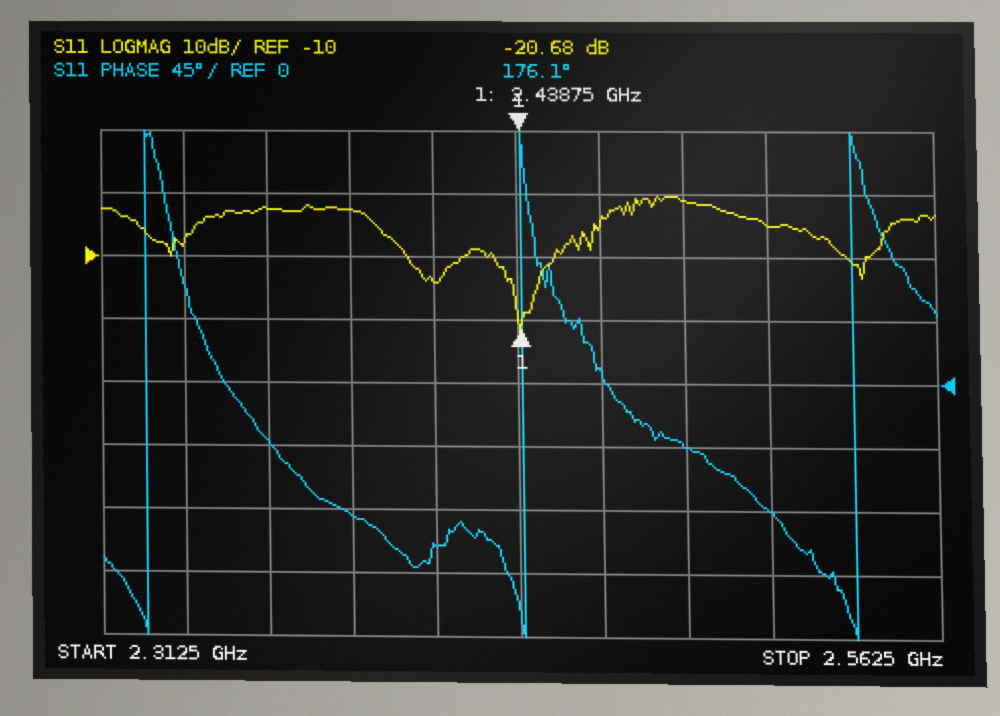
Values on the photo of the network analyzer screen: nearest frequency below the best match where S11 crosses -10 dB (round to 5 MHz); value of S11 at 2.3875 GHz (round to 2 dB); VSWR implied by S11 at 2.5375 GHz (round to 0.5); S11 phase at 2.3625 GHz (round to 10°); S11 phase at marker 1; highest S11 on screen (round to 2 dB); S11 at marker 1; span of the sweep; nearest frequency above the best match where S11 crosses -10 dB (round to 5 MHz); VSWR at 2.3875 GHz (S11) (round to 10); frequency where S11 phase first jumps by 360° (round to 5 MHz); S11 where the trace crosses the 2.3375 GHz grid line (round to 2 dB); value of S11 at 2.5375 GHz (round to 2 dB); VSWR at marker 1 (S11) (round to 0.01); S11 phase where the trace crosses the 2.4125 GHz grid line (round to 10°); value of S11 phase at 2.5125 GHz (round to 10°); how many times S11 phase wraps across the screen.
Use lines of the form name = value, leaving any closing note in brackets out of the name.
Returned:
nearest frequency below the best match where S11 crosses -10 dB = 2.430 GHz
value of S11 at 2.3875 GHz = -2 dB
VSWR implied by S11 at 2.5375 GHz = 2.0
S11 phase at 2.3625 GHz = -40°
S11 phase at marker 1 = 176.1°
highest S11 on screen = 0 dB
S11 at marker 1 = -20.68 dB
span of the sweep = 250 MHz
nearest frequency above the best match where S11 crosses -10 dB = 2.450 GHz
VSWR at 2.3875 GHz (S11) = 10
frequency where S11 phase first jumps by 360° = 2.325 GHz
S11 where the trace crosses the 2.3375 GHz grid line = -8 dB
value of S11 at 2.5375 GHz = -10 dB
VSWR at marker 1 (S11) = 1.20
S11 phase where the trace crosses the 2.4125 GHz grid line = -120°
value of S11 phase at 2.5125 GHz = -90°
how many times S11 phase wraps across the screen = 3
